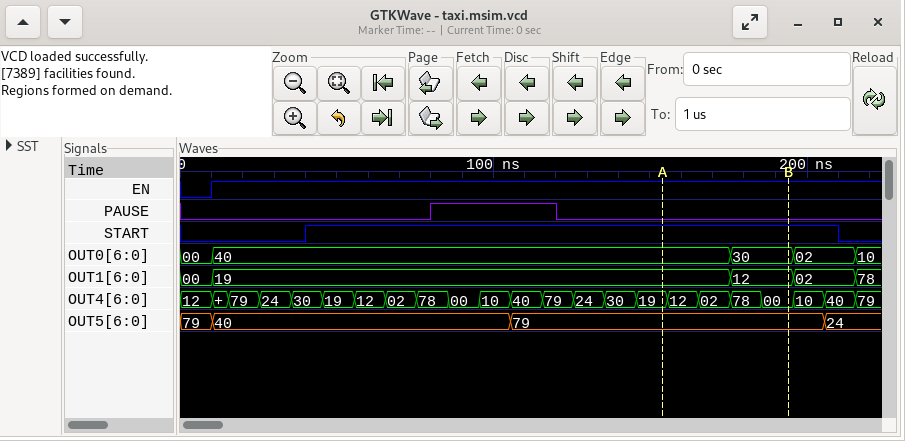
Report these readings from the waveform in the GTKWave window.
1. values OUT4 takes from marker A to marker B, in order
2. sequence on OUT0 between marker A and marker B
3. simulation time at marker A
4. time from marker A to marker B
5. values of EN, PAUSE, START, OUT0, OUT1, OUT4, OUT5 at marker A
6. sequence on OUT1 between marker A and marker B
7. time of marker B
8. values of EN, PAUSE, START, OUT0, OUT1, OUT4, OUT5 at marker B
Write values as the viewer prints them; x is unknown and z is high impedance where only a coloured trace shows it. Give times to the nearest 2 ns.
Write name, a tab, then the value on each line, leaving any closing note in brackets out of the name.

values OUT4 takes from marker A to marker B, in order	19, 12, 02, 78, 00
sequence on OUT0 between marker A and marker B	40, 30
simulation time at marker A	154 ns
time from marker A to marker B	40 ns
values of EN, PAUSE, START, OUT0, OUT1, OUT4, OUT5 at marker A	EN=1, PAUSE=0, START=1, OUT0=40, OUT1=19, OUT4=19, OUT5=79
sequence on OUT1 between marker A and marker B	19, 12
time of marker B	194 ns
values of EN, PAUSE, START, OUT0, OUT1, OUT4, OUT5 at marker B	EN=1, PAUSE=0, START=1, OUT0=30, OUT1=12, OUT4=00, OUT5=79
